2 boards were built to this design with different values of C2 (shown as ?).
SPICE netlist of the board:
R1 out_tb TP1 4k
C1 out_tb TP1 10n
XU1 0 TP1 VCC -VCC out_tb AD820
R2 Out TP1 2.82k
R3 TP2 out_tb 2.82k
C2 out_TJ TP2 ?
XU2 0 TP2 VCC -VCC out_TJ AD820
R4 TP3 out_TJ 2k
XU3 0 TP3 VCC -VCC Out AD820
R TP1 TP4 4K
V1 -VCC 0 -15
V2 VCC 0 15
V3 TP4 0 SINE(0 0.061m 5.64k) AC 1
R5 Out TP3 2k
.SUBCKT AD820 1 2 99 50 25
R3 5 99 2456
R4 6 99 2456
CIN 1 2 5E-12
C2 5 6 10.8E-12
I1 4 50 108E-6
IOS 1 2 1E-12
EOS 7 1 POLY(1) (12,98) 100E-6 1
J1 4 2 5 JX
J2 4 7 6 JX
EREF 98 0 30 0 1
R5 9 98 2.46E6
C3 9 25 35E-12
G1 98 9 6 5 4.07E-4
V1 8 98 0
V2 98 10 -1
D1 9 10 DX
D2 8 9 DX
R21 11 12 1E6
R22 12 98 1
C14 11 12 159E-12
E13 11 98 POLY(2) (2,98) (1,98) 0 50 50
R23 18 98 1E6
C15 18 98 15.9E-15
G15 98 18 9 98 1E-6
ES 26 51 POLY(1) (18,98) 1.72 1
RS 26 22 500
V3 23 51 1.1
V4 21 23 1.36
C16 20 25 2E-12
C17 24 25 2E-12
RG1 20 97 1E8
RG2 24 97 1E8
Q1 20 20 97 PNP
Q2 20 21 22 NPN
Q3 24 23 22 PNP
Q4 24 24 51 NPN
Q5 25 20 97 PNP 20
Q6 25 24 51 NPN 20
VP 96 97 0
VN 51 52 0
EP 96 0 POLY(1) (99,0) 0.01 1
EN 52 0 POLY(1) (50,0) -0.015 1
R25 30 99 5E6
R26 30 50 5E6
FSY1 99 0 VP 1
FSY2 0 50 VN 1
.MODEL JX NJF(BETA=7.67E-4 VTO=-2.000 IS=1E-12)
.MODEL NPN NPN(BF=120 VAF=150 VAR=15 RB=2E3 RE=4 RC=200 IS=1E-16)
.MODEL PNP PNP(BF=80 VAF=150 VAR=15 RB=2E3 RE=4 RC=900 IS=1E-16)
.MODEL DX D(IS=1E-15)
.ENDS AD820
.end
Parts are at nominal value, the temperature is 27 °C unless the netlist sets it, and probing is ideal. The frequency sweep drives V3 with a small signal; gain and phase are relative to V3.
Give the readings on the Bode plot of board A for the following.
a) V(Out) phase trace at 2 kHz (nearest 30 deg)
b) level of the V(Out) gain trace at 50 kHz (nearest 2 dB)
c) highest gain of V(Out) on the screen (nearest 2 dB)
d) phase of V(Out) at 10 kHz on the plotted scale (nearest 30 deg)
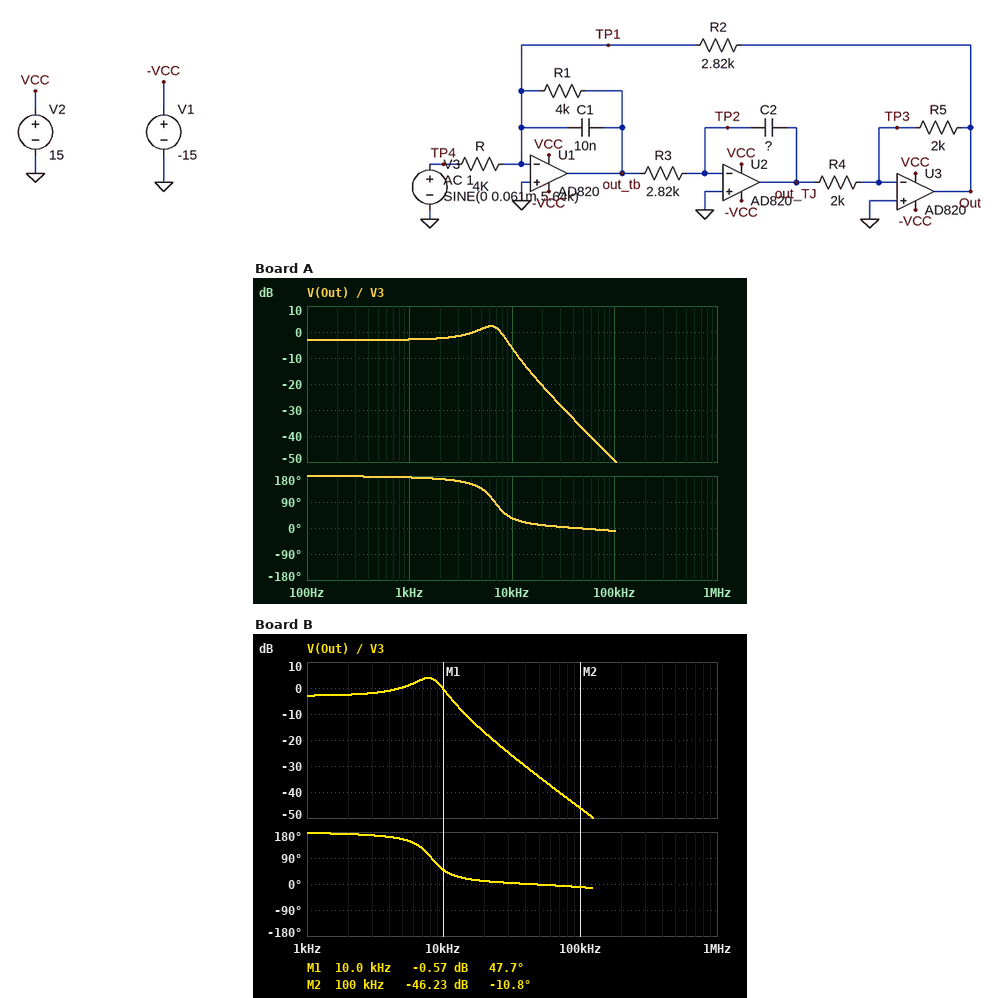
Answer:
180 deg
-38 dB
2 dB
30 deg
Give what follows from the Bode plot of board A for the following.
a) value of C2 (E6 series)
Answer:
6.8 nF
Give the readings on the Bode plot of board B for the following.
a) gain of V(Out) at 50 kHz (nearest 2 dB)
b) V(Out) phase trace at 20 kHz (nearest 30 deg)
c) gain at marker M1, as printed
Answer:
-34 dB
0 deg
-0.57 dB
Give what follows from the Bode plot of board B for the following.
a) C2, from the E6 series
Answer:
4.7 nF
